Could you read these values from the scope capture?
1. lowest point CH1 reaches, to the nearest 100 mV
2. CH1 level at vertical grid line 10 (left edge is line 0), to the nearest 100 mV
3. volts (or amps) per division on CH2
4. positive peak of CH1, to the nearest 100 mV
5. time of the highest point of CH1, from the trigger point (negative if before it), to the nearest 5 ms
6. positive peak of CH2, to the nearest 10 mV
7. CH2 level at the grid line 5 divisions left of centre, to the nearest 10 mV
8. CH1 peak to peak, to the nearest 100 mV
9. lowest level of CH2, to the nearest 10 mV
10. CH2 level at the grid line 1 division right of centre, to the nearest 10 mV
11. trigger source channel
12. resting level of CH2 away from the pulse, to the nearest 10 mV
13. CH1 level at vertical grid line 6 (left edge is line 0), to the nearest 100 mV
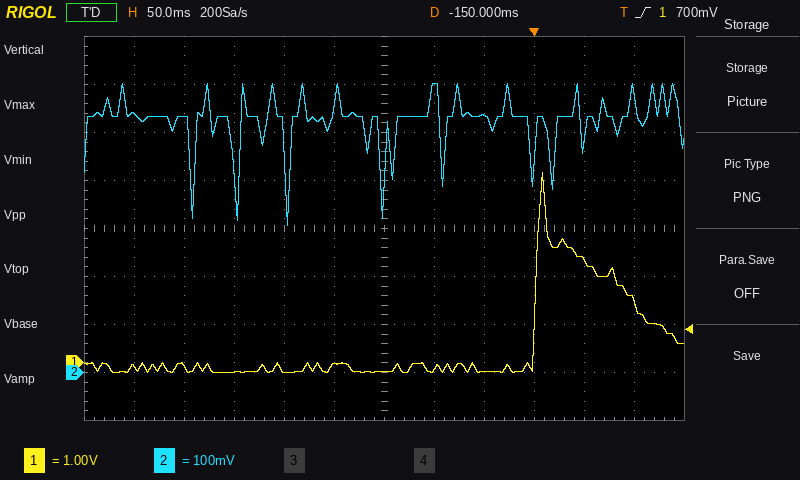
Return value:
-200 mV
2.1 V
100 mV
4.0 V
+10 ms
600 mV
540 mV
4.2 V
310 mV
590 mV
CH1
530 mV
-200 mV
